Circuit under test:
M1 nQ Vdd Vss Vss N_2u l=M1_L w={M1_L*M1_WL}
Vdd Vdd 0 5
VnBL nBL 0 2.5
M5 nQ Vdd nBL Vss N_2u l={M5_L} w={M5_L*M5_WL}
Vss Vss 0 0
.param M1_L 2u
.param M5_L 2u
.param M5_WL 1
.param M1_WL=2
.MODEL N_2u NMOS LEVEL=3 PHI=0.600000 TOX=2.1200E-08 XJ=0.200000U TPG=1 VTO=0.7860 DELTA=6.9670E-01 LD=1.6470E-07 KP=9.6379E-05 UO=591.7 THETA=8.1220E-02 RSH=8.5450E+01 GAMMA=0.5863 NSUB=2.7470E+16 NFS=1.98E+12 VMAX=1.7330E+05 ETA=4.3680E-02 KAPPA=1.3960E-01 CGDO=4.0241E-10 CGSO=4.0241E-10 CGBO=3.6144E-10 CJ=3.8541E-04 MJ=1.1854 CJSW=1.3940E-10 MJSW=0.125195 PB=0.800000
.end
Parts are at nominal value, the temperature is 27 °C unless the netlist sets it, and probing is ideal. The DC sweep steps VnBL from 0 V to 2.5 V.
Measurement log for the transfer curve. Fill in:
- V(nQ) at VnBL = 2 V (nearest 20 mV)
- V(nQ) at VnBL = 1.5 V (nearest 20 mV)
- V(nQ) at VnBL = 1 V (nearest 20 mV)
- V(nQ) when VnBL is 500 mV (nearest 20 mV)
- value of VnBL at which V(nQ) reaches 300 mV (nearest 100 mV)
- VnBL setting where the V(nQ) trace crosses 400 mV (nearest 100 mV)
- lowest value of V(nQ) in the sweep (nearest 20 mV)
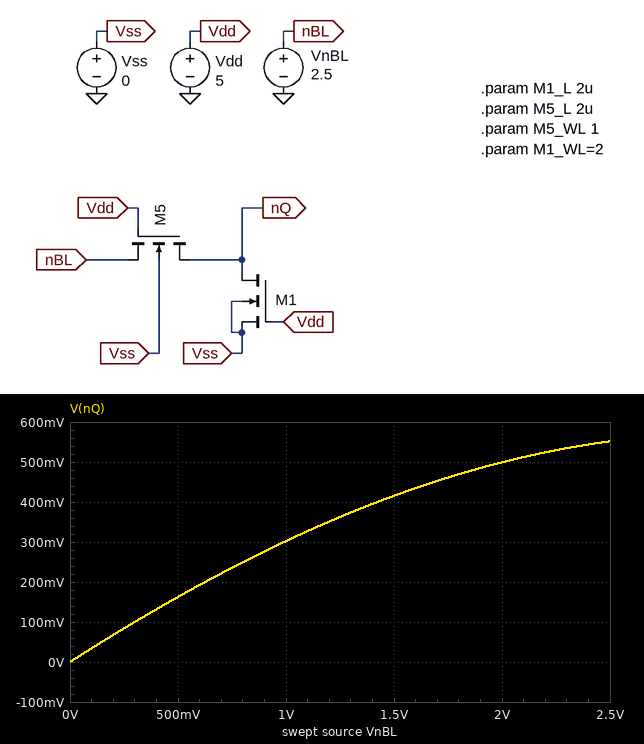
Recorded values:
500 mV
420 mV
300 mV
160 mV
1.0 V
1.4 V
0 V
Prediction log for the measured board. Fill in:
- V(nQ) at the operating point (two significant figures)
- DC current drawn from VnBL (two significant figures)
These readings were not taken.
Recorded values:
550 mV
310 µA
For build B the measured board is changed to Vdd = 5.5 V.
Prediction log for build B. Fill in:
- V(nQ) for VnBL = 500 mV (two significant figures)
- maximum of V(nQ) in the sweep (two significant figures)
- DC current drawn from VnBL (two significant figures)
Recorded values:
160 mV
590 mV
360 µA
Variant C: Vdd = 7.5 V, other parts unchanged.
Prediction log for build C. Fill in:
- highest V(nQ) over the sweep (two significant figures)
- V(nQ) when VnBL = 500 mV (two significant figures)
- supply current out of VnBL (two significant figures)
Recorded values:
690 mV
170 mV
520 µA
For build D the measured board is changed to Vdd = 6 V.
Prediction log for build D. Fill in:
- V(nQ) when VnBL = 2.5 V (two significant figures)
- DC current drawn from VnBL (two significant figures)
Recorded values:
620 mV
400 µA
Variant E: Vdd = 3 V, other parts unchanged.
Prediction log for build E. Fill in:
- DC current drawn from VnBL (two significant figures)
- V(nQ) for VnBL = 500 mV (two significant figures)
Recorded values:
110 µA
150 mV
